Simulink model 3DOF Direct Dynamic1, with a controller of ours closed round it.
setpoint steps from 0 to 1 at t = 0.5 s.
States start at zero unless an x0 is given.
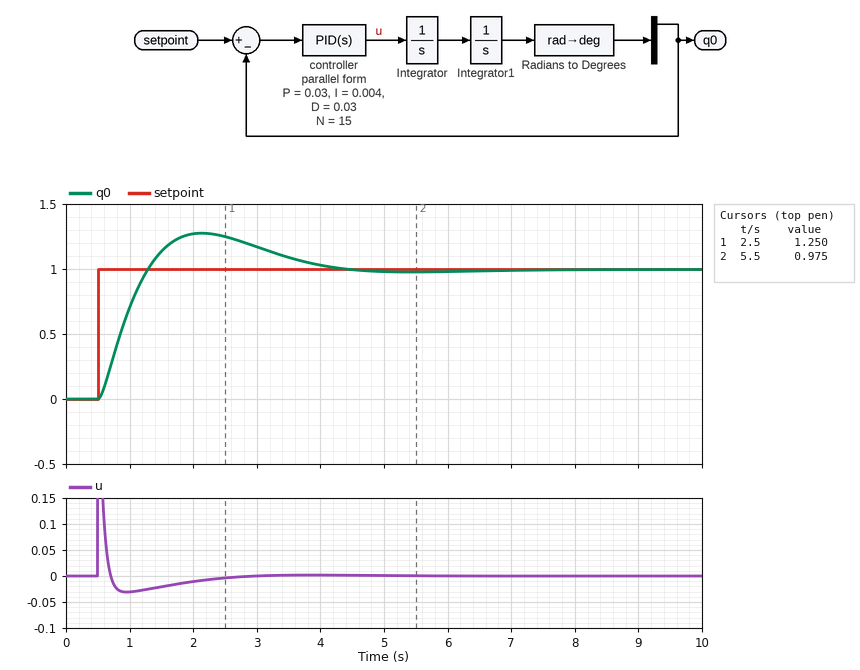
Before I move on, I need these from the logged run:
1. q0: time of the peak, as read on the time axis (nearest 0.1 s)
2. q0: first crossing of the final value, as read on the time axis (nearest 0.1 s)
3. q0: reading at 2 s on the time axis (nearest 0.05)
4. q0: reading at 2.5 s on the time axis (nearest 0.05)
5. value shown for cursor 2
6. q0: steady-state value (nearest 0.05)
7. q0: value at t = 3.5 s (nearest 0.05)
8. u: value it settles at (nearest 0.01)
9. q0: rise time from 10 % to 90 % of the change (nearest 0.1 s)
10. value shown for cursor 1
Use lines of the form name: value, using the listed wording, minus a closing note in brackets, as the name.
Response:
q0: time of the peak, as read on the time axis: 2.1 s
q0: first crossing of the final value, as read on the time axis: 1.3 s
q0: reading at 2 s on the time axis: 1.25
q0: reading at 2.5 s on the time axis: 1.25
value shown for cursor 2: 0.975
q0: steady-state value: 1.00
q0: value at t = 3.5 s: 1.10
u: value it settles at: 0.00
q0: rise time from 10 % to 90 % of the change: 0.6 s
value shown for cursor 1: 1.250
